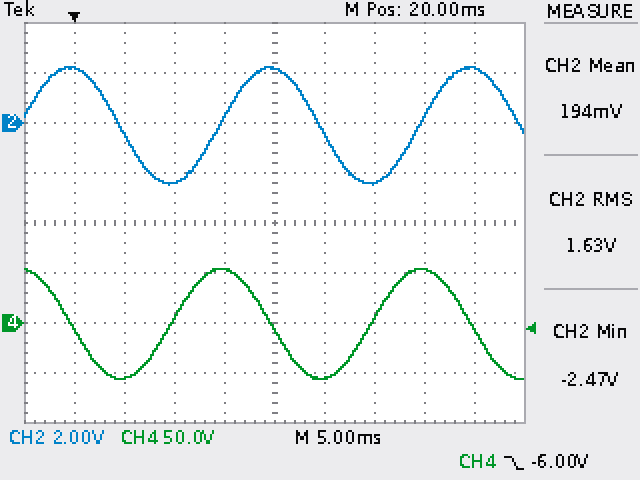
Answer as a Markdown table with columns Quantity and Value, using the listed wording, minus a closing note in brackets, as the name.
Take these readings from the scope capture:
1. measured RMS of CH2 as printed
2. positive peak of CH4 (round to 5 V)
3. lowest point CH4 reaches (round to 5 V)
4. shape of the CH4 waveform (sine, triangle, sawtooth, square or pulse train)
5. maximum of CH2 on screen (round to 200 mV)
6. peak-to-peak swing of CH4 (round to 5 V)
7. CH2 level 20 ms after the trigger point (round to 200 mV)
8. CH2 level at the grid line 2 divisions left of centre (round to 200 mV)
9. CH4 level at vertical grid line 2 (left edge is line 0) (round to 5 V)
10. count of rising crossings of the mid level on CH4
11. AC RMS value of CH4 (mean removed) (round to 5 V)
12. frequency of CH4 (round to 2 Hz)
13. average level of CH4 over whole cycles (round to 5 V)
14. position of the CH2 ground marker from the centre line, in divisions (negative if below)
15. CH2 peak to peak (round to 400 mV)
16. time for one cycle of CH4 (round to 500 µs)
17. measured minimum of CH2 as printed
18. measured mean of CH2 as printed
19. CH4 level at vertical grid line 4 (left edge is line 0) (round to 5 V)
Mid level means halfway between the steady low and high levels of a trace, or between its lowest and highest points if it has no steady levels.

| Quantity | Value |
|---|---|
| measured RMS of CH2 as printed | 1.63 V |
| positive peak of CH4 | 55 V |
| lowest point CH4 reaches | -55 V |
| shape of the CH4 waveform | sine |
| maximum of CH2 on screen | 2.2 V |
| peak-to-peak swing of CH4 | 110 V |
| CH2 level 20 ms after the trigger point | 2.2 V |
| CH2 level at the grid line 2 divisions left of centre | -2.4 V |
| CH4 level at vertical grid line 2 (left edge is line 0) | -55 V |
| count of rising crossings of the mid level on CH4 | 2 |
| AC RMS value of CH4 (mean removed) | 40 V |
| frequency of CH4 | 50 Hz |
| average level of CH4 over whole cycles | 0 V |
| position of the CH2 ground marker from the centre line, in divisions | +2.0 div |
| CH2 peak to peak | 4.8 V |
| time for one cycle of CH4 | 20.0 ms |
| measured minimum of CH2 as printed | -2.47 V |
| measured mean of CH2 as printed | 194 mV |
| CH4 level at vertical grid line 4 (left edge is line 0) | 55 V |
